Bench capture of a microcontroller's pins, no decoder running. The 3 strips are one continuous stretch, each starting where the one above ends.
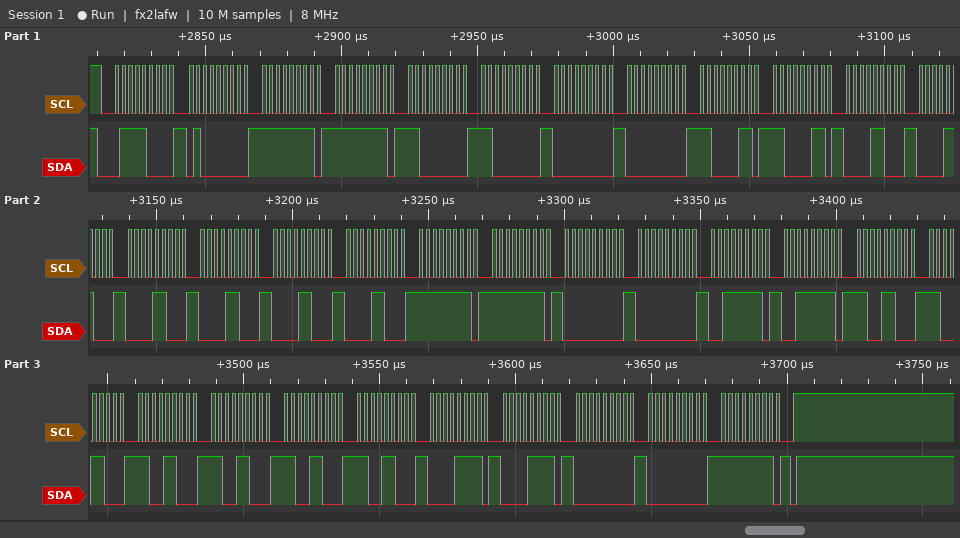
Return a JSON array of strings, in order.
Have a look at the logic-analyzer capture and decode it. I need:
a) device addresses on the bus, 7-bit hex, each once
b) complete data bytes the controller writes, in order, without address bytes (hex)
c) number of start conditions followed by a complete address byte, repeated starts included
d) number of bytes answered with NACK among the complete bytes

["0x3C", "40 FF FF C0 C0 00 00 C3 C3 0C 0C 0C 0C 0C 0C FF FF 00 00 3F 3F CC CC CC CC CC CC 0F 0F 00 00 FF", "1", "0"]
